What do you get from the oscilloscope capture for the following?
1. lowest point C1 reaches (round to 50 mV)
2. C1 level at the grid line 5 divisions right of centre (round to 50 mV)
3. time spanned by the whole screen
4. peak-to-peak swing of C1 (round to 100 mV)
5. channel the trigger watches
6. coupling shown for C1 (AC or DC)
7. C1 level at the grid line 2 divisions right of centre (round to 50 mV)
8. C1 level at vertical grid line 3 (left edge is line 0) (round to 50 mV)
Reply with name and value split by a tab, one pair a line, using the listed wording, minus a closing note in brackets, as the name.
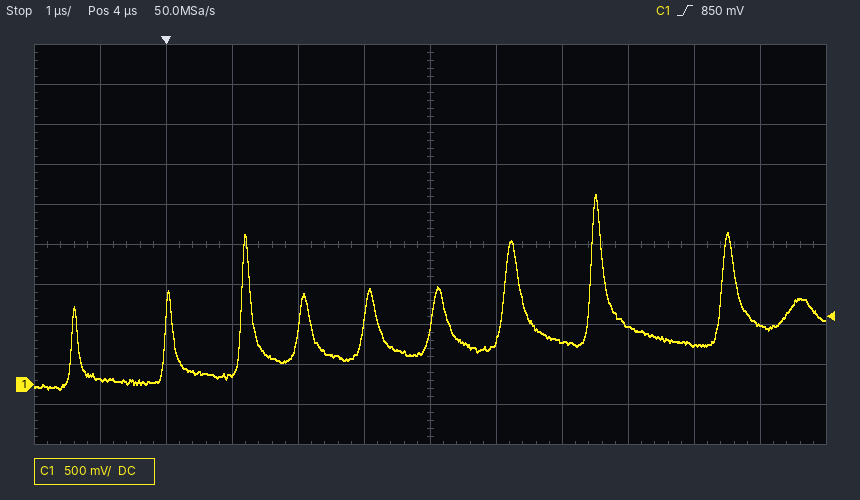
lowest point C1 reaches	-50 mV
C1 level at the grid line 5 divisions right of centre	750 mV
time spanned by the whole screen	12 µs
peak-to-peak swing of C1	2.40 V
channel the trigger watches	C1
coupling shown for C1	DC
C1 level at the grid line 2 divisions right of centre	550 mV
C1 level at vertical grid line 3 (left edge is line 0)	150 mV
